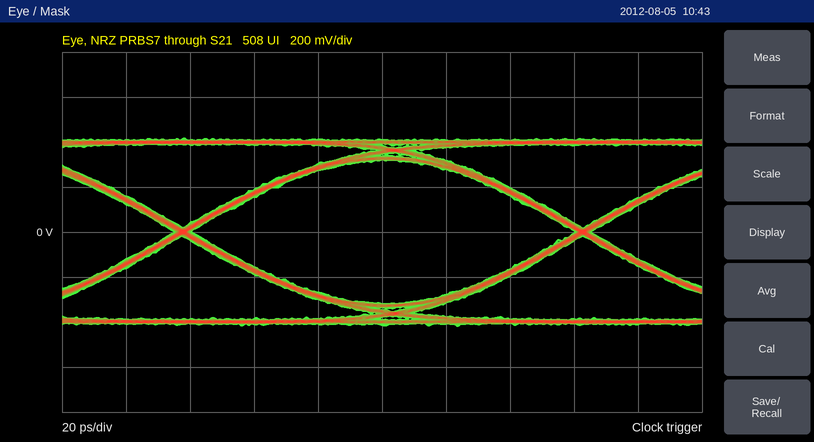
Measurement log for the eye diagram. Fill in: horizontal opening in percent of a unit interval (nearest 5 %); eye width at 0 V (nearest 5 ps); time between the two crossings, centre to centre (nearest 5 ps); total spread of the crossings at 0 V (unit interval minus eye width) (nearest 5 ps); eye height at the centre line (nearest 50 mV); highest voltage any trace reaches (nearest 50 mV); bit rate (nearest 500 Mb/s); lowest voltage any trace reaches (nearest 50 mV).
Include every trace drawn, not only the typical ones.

95 %
120 ps
125 ps
5 ps
650 mV
400 mV
8.0 Gb/s
-400 mV
